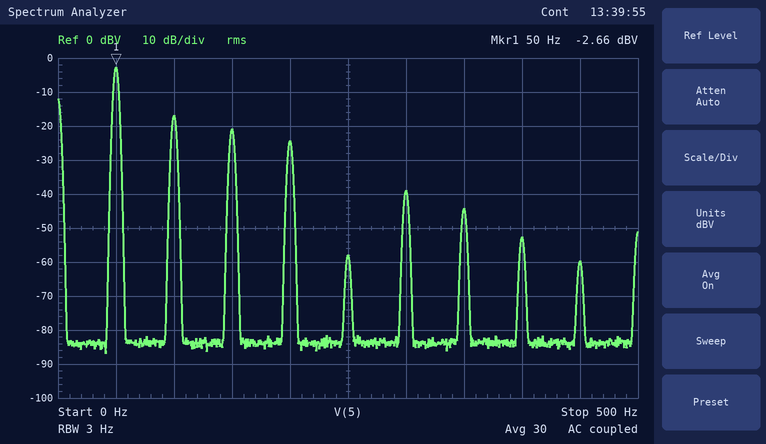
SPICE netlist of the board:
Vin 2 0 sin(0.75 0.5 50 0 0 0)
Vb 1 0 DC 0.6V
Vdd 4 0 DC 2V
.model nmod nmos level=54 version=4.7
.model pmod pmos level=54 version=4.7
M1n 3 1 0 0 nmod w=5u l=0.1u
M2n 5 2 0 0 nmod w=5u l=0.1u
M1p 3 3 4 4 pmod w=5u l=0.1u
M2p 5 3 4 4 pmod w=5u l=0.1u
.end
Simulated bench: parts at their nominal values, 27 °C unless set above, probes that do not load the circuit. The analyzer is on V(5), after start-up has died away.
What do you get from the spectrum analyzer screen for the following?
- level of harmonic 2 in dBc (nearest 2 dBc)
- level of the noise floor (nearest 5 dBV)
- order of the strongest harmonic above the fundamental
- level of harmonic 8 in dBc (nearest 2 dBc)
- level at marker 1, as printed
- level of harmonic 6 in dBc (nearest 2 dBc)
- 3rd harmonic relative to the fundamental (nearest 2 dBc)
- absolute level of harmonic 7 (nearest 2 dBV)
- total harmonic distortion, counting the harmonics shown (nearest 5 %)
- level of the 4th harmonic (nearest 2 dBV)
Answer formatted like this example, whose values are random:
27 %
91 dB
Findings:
-14 dBc
-85 dBV
2
-50 dBc
-2.66 dBV
-36 dBc
-18 dBc
-44 dBV
25 %
-24 dBV
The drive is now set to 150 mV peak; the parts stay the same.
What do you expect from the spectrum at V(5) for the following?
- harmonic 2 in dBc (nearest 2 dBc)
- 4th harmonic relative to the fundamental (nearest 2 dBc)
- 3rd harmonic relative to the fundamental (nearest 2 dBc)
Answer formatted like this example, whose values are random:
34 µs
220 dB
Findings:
-18 dBc
-60 dBc
-44 dBc
